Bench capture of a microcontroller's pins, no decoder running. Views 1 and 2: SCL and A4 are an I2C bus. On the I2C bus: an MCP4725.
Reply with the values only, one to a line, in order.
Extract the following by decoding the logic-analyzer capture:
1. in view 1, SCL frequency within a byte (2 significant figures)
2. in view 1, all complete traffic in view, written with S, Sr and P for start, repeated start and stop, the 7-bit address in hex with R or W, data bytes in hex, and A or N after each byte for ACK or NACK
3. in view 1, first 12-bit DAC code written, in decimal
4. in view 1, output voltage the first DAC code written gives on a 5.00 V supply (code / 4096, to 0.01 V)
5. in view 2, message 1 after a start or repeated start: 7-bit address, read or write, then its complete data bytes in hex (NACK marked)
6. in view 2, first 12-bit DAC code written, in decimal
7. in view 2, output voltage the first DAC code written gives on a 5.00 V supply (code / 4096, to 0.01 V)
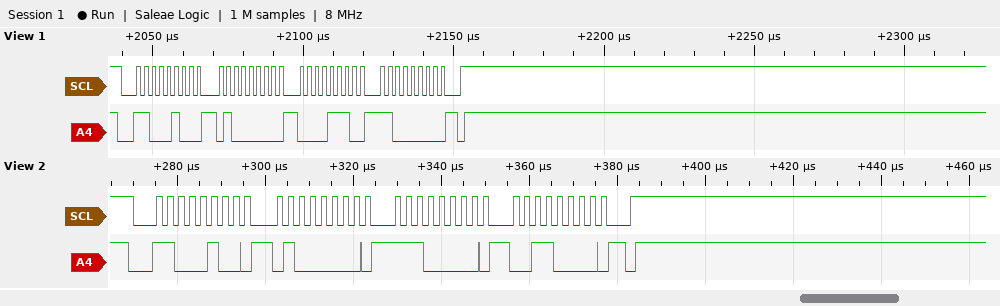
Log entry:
400 kHz
S 62W A 40 A 0E A C0 A P
236
0.29 V
0x62 write: 40 E0 30
3587
4.38 V
